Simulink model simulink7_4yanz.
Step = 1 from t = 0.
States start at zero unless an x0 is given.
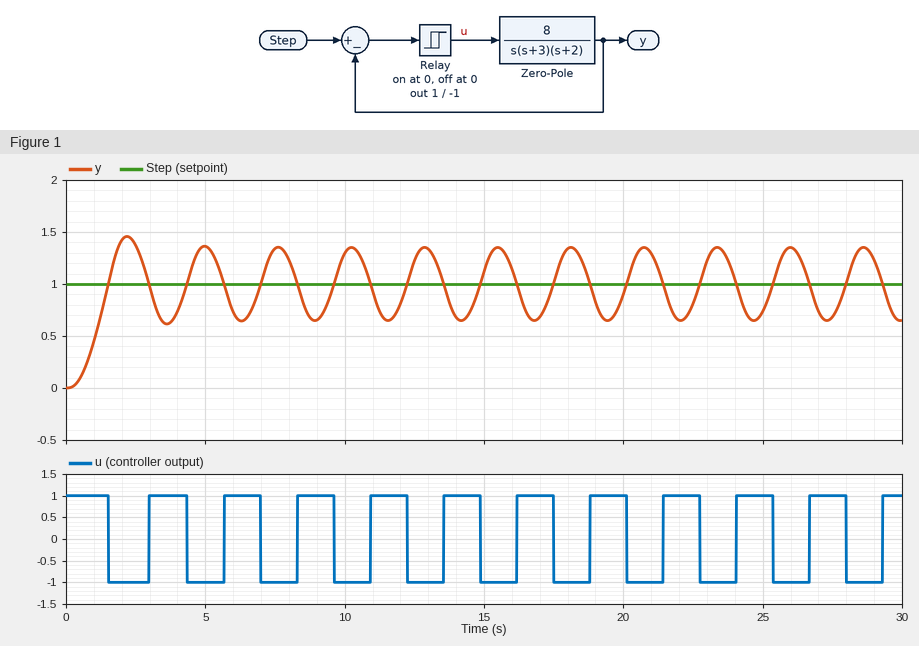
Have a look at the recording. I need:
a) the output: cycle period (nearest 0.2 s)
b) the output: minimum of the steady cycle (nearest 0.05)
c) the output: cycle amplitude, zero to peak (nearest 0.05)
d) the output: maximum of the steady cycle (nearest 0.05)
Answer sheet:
2.6 s
0.65
0.35
1.35
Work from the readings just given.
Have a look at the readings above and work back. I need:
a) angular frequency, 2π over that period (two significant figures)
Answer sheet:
2.4 rad/s
